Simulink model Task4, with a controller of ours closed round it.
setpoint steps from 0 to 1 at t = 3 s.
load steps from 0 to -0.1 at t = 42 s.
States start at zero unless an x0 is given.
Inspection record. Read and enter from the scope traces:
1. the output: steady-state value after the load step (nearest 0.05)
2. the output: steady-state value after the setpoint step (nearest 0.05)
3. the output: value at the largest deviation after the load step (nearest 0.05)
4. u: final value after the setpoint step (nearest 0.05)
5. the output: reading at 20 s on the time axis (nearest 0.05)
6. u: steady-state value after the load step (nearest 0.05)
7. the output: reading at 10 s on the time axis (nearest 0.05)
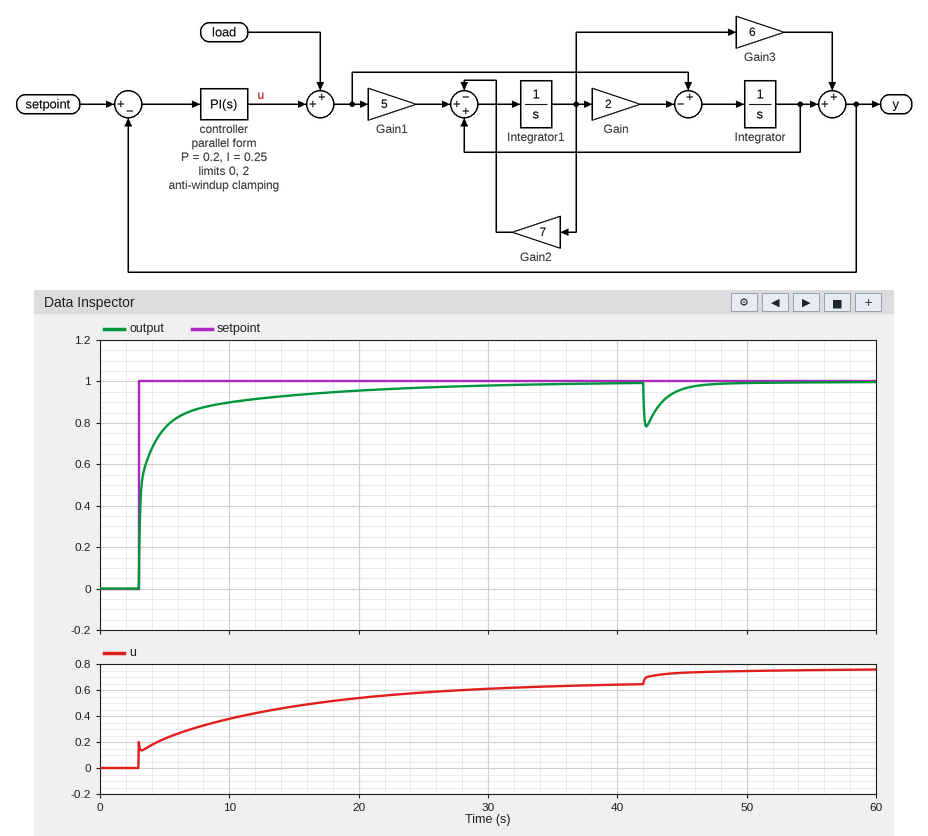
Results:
1.00
1.00
0.80
0.65
0.95
0.75
0.90
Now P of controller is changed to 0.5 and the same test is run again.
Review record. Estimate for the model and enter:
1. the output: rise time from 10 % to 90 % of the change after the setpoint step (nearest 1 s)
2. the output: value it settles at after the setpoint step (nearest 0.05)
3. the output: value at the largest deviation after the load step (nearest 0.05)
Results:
8 s
1.00
0.85
